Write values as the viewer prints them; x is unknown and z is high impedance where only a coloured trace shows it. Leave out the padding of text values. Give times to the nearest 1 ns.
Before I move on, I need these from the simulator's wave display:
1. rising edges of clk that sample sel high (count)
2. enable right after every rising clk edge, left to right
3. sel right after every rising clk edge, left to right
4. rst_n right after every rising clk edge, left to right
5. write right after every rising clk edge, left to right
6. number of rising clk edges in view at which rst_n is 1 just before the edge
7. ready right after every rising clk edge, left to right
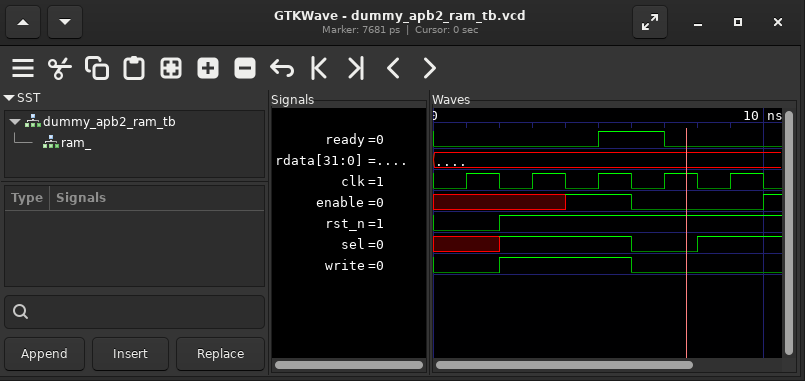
3
x x 1 0 0
x 1 1 0 1
0 1 1 1 1
0 1 1 0 0
4
0 0 1 0 0
